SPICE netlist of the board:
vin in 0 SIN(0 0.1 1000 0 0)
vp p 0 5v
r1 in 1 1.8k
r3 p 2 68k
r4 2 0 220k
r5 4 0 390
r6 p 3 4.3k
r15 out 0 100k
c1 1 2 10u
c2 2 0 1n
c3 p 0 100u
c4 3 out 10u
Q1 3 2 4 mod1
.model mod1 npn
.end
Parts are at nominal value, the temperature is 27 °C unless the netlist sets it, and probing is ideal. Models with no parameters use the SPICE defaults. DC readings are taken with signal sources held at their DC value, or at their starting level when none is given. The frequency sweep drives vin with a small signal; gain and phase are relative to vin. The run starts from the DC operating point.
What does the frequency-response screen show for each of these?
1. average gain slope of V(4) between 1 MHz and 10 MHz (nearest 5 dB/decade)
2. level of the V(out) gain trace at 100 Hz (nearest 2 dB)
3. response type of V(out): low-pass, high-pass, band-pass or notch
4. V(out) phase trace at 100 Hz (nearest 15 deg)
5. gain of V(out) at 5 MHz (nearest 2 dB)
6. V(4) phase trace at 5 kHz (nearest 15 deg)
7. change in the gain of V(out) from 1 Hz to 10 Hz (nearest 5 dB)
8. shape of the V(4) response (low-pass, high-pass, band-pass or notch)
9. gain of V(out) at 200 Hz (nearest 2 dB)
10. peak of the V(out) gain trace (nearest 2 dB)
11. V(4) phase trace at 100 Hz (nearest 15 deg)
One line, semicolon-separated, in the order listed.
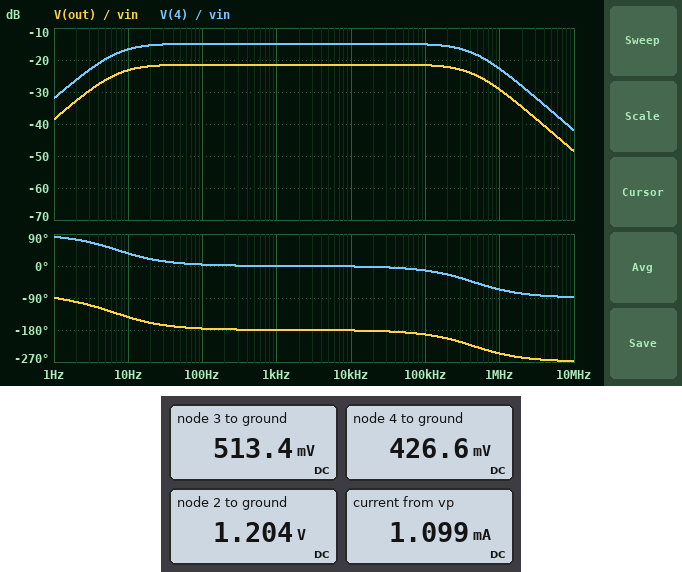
-20 dB/decade; -22 dB; band-pass; -180 deg; -42 dB; 0 deg; 15 dB; band-pass; -22 dB; -22 dB; 0 deg
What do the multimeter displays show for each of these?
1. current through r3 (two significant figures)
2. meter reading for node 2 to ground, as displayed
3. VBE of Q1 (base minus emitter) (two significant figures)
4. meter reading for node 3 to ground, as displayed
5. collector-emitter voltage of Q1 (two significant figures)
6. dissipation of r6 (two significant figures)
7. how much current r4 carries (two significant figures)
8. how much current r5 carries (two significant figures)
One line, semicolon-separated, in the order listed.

56 µA; 1.204 V; 780 mV; 513.4 mV; 87 mV; 4.7 mW; 5.5 µA; 1.1 mA
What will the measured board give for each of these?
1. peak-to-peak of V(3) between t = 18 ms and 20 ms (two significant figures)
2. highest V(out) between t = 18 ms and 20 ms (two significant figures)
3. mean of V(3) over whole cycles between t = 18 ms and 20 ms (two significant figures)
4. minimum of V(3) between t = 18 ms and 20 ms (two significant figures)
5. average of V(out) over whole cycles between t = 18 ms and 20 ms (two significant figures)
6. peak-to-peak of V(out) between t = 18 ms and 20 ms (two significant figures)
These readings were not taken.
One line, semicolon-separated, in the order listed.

110 mV; 110 mV; 530 mV; 510 mV; 18 mV; 110 mV
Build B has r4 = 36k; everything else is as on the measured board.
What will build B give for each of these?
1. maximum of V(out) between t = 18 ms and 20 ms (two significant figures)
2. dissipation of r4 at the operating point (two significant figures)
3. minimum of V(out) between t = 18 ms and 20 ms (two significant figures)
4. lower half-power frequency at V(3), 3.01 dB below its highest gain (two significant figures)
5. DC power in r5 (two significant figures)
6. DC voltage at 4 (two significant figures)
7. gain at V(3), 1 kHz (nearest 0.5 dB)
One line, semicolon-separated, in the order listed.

720 mV; 39 µW; -21 mV; 6.7 Hz; 440 µW; 410 mV; -4.5 dB
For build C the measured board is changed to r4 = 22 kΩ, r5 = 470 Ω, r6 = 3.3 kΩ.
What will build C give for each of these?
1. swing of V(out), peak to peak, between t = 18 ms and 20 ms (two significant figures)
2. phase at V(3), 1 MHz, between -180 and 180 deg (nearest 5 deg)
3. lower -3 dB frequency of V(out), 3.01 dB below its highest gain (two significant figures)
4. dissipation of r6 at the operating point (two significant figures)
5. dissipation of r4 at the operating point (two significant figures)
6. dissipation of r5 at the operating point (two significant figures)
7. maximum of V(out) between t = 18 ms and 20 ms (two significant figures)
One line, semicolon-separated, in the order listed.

1.1 V; 95 deg; 1.1 Hz; 1.7 mW; 55 µW; 240 µW; 540 mV
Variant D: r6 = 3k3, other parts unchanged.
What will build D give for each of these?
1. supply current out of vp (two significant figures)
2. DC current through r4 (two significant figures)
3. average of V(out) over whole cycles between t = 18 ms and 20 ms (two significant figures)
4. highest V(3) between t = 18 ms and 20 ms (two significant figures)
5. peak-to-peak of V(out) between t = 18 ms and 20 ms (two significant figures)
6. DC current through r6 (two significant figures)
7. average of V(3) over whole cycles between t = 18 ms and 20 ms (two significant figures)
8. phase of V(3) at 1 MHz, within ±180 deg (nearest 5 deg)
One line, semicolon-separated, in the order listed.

1.4 mA; 6.0 µA; 30 mV; 800 mV; 180 mV; 1.3 mA; 660 mV; 115 deg
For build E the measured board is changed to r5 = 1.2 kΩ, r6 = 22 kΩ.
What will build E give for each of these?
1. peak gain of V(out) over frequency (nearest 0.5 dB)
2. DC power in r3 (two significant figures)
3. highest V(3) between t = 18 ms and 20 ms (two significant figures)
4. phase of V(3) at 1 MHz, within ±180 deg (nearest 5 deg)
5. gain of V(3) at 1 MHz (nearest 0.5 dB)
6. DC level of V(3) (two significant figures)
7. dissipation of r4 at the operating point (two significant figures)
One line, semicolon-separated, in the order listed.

-12.0 dB; 230 µW; 390 mV; -80 deg; -25.5 dB; 360 mV; 5.1 µW
